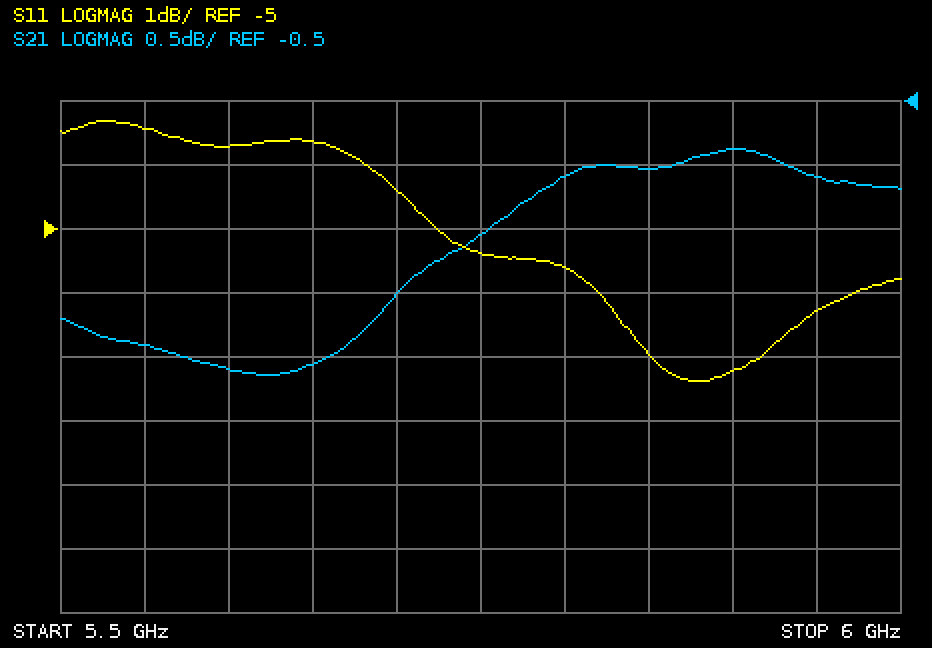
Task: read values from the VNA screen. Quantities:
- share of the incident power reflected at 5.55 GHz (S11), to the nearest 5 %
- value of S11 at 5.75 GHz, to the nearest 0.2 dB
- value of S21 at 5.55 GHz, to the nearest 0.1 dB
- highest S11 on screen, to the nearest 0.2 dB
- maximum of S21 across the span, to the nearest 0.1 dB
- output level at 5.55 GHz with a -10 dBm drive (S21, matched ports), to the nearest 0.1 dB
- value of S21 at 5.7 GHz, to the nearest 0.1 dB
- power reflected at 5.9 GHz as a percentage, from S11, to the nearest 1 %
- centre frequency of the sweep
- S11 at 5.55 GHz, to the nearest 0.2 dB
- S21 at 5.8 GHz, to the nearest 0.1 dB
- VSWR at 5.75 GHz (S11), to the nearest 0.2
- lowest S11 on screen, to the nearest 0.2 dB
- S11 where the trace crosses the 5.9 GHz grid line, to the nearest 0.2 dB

45 %
-5.4 dB
-2.4 dB
-3.4 dB
-0.9 dB
-12.4 dBm
-2.0 dB
19 %
5.75 GHz
-3.4 dB
-1.1 dB
3.4
-7.4 dB
-7.2 dB
